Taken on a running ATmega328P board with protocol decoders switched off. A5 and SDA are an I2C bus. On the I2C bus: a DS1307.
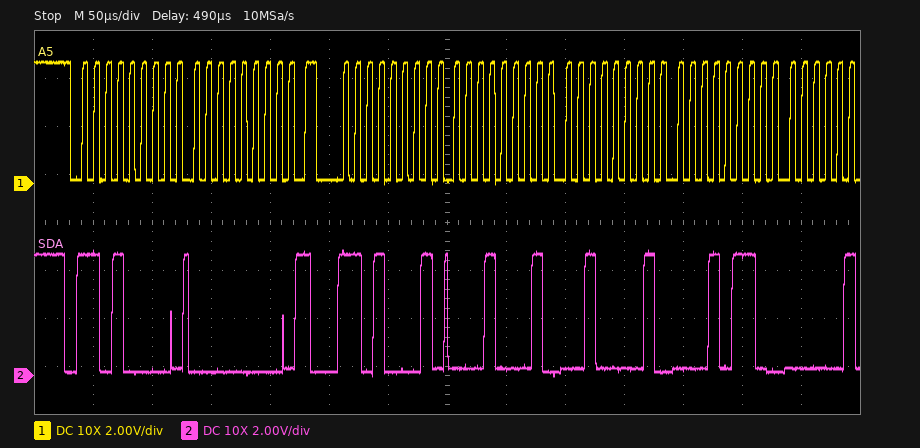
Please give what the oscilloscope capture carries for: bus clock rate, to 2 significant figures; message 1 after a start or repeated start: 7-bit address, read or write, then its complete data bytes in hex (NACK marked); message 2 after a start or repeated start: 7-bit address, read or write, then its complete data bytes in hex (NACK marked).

100 kHz
0x68 write: 00
0x68 read: 11 21 16
